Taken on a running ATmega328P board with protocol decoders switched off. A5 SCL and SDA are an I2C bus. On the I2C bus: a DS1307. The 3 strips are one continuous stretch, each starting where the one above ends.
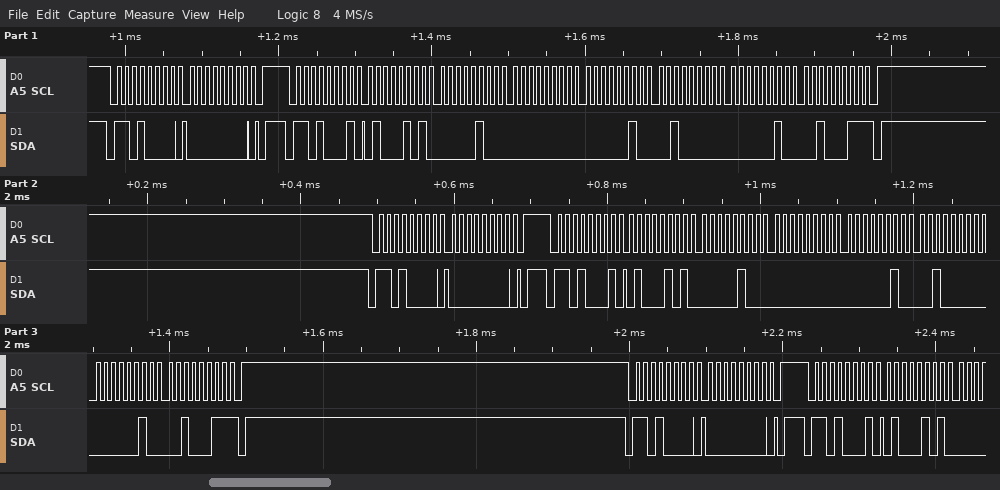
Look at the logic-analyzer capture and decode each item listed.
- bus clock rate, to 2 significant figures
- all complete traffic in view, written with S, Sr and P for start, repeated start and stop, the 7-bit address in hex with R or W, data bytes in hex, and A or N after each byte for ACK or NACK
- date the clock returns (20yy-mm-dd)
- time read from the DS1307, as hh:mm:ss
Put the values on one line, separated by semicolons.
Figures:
100 kHz; S 68W A 00 A P S 68R A 45 A 04 A 00 A 02 A 20 A 02 A 23 N P S 68W A 00 A P S 68R A 45 A 04 A 00 A 02 A 20 A 02 A 23 N P S 68W A 00 A P S 68R A 45 A; 2023-02-20; 00:04:45
